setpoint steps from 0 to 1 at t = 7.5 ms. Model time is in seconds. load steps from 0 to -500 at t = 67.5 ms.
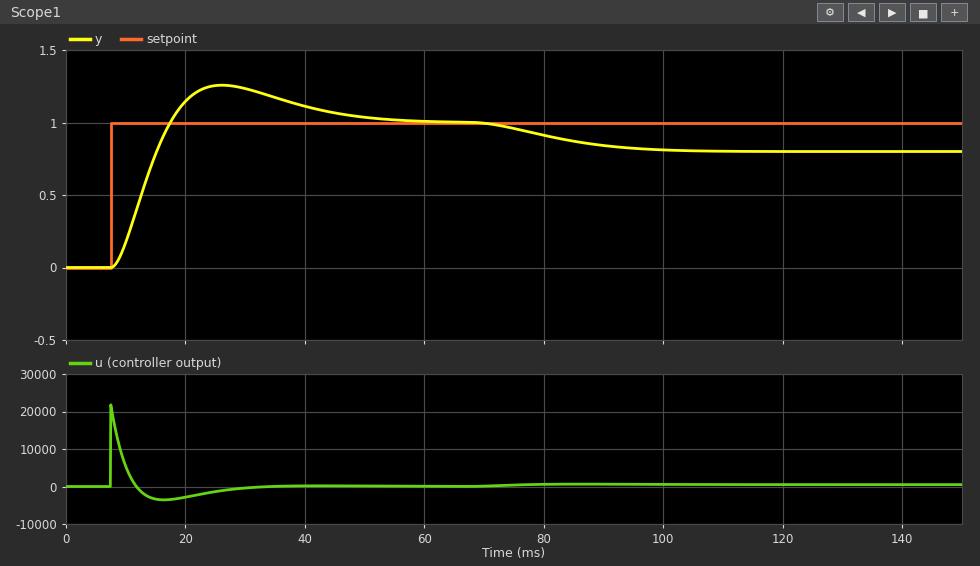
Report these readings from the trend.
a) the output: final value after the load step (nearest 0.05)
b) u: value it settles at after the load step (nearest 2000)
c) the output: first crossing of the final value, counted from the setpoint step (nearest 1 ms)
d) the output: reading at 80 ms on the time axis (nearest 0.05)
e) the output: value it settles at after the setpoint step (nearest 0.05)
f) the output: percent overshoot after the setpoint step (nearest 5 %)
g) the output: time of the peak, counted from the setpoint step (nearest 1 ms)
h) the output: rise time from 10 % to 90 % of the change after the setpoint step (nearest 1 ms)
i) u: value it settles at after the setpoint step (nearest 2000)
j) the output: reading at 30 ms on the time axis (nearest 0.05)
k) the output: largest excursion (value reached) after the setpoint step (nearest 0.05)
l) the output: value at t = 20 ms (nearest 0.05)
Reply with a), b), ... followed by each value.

a) 0.80
b) 0
c) 10 ms
d) 0.90
e) 1.00
f) 25 %
g) 19 ms
h) 7 ms
i) 0
j) 1.25
k) 1.25
l) 1.15
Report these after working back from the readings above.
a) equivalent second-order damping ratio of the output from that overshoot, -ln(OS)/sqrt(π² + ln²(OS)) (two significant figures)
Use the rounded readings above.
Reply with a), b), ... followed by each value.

a) 0.40
